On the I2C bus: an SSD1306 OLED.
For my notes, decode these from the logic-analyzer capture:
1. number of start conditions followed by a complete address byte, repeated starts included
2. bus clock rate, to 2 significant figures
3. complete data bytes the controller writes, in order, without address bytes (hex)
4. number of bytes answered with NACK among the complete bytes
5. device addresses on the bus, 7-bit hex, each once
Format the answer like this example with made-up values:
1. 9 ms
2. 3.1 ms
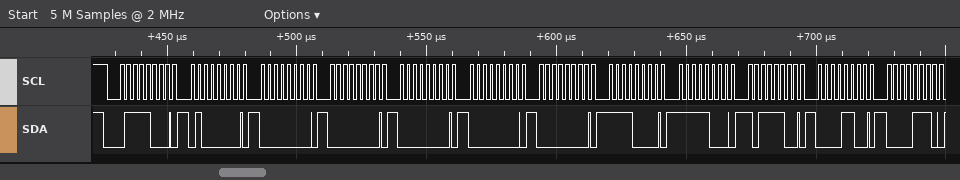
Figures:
1. 1
2. 400 kHz
3. 40 00 00 00 00 00 F0 F8 BC 0C 0E
4. 0
5. 0x3C
